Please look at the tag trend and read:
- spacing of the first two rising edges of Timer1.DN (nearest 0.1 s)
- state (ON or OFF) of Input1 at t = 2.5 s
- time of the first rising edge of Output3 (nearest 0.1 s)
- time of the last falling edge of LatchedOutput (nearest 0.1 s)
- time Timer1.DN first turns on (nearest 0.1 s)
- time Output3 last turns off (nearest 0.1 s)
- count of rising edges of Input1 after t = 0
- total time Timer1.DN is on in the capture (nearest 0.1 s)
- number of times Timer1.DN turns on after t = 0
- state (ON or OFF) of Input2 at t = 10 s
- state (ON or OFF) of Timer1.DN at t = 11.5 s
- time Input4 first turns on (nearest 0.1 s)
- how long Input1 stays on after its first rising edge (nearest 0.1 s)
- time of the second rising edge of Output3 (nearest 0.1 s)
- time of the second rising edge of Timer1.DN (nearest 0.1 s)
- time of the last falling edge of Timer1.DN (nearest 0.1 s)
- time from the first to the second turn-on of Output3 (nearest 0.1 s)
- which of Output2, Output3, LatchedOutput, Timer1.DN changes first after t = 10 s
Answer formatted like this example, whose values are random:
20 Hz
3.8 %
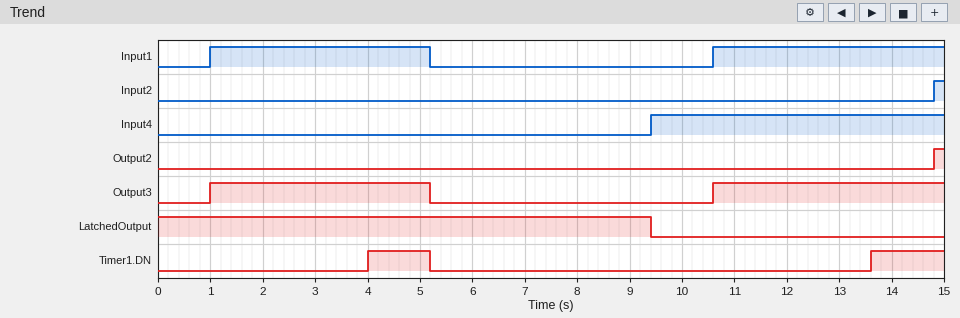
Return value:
9.6 s
ON
1.0 s
9.4 s
4.0 s
5.2 s
2
2.6 s
2
OFF
OFF
9.4 s
4.2 s
10.6 s
13.6 s
5.2 s
9.6 s
Output3
